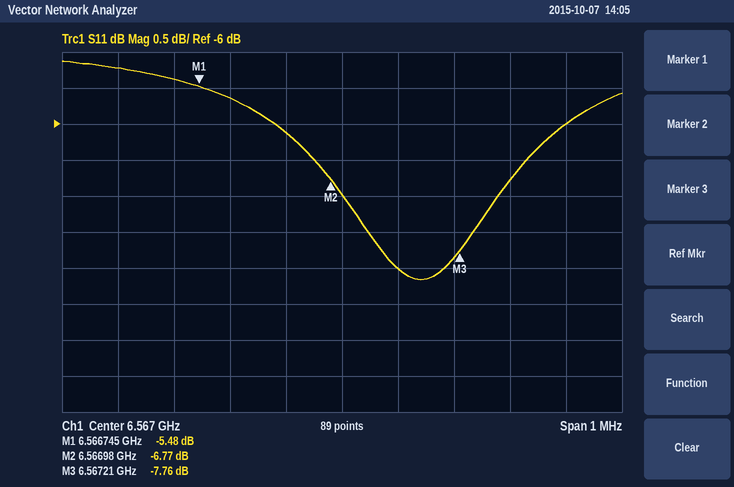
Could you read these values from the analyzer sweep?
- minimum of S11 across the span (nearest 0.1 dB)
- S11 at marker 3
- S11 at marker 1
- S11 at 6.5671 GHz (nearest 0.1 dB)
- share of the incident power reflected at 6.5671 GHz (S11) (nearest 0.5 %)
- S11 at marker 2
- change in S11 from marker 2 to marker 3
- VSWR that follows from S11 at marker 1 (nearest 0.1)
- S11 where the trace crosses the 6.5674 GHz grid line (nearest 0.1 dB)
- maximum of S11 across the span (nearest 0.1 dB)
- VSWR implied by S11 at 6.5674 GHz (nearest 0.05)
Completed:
-8.2 dB
-7.76 dB
-5.48 dB
-8.0 dB
16.0 %
-6.77 dB
-0.99 dB
3.3
-6.0 dB
-5.1 dB
3.00
